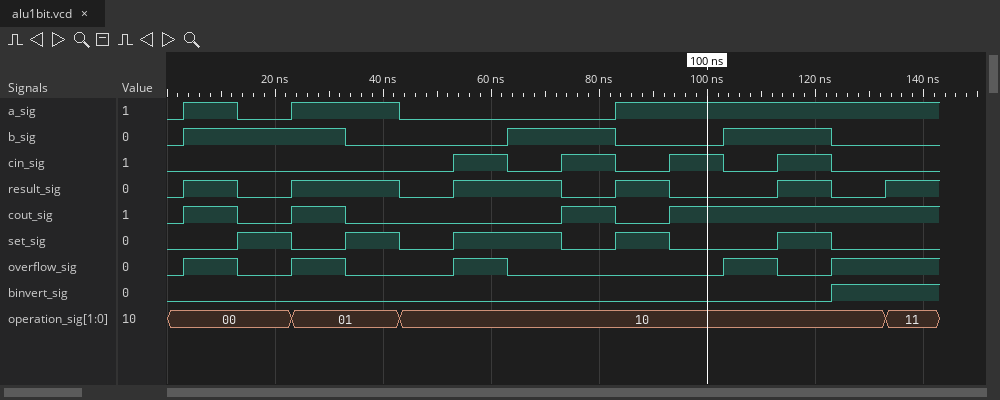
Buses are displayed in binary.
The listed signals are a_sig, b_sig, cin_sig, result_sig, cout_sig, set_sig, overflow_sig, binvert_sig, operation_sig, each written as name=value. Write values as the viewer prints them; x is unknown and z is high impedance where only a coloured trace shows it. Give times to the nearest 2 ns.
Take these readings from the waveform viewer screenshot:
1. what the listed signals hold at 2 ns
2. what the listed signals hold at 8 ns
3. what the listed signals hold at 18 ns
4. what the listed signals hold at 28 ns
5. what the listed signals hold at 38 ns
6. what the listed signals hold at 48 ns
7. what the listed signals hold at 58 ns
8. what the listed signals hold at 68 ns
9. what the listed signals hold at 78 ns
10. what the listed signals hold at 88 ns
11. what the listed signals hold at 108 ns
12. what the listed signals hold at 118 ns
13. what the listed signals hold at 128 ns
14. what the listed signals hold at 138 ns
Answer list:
a_sig=0, b_sig=0, cin_sig=0, result_sig=0, cout_sig=0, set_sig=0, overflow_sig=0, binvert_sig=0, operation_sig=00
a_sig=1, b_sig=1, cin_sig=0, result_sig=1, cout_sig=1, set_sig=0, overflow_sig=1, binvert_sig=0, operation_sig=00
a_sig=0, b_sig=1, cin_sig=0, result_sig=0, cout_sig=0, set_sig=1, overflow_sig=0, binvert_sig=0, operation_sig=00
a_sig=1, b_sig=1, cin_sig=0, result_sig=1, cout_sig=1, set_sig=0, overflow_sig=1, binvert_sig=0, operation_sig=01
a_sig=1, b_sig=0, cin_sig=0, result_sig=1, cout_sig=0, set_sig=1, overflow_sig=0, binvert_sig=0, operation_sig=01
a_sig=0, b_sig=0, cin_sig=0, result_sig=0, cout_sig=0, set_sig=0, overflow_sig=0, binvert_sig=0, operation_sig=10
a_sig=0, b_sig=0, cin_sig=1, result_sig=1, cout_sig=0, set_sig=1, overflow_sig=1, binvert_sig=0, operation_sig=10
a_sig=0, b_sig=1, cin_sig=0, result_sig=1, cout_sig=0, set_sig=1, overflow_sig=0, binvert_sig=0, operation_sig=10
a_sig=0, b_sig=1, cin_sig=1, result_sig=0, cout_sig=1, set_sig=0, overflow_sig=0, binvert_sig=0, operation_sig=10
a_sig=1, b_sig=0, cin_sig=0, result_sig=1, cout_sig=0, set_sig=1, overflow_sig=0, binvert_sig=0, operation_sig=10
a_sig=1, b_sig=1, cin_sig=0, result_sig=0, cout_sig=1, set_sig=0, overflow_sig=1, binvert_sig=0, operation_sig=10
a_sig=1, b_sig=1, cin_sig=1, result_sig=1, cout_sig=1, set_sig=1, overflow_sig=0, binvert_sig=0, operation_sig=10
a_sig=1, b_sig=0, cin_sig=0, result_sig=0, cout_sig=1, set_sig=0, overflow_sig=1, binvert_sig=1, operation_sig=10
a_sig=1, b_sig=0, cin_sig=0, result_sig=1, cout_sig=1, set_sig=0, overflow_sig=1, binvert_sig=1, operation_sig=11
